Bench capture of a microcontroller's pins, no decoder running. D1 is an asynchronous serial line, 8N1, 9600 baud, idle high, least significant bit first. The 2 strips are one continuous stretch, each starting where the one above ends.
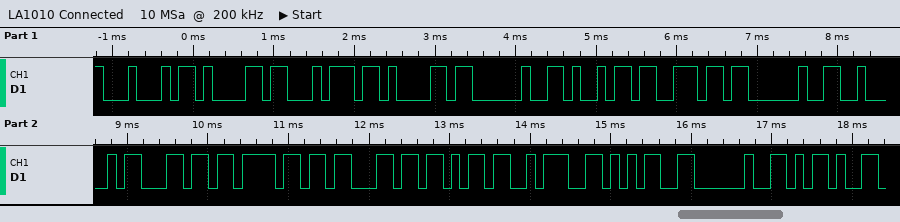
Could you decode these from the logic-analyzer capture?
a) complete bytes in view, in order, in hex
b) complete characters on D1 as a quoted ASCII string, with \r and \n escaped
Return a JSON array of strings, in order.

["44 61 74 61 20 69 6E 20 42 6C 6F 63 6B 3A 35 20 2D", "\"Data in Block:5 -\""]
